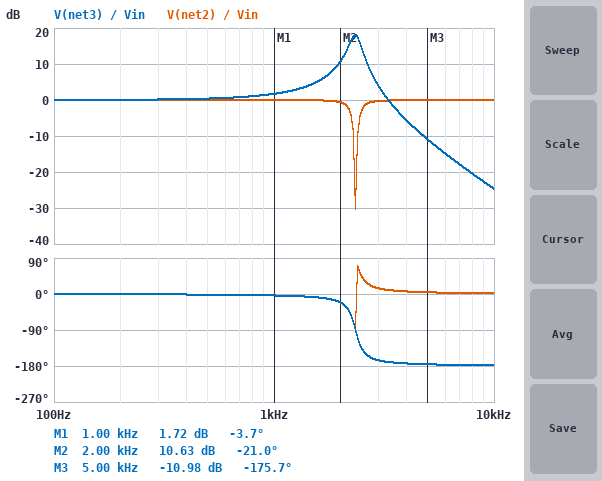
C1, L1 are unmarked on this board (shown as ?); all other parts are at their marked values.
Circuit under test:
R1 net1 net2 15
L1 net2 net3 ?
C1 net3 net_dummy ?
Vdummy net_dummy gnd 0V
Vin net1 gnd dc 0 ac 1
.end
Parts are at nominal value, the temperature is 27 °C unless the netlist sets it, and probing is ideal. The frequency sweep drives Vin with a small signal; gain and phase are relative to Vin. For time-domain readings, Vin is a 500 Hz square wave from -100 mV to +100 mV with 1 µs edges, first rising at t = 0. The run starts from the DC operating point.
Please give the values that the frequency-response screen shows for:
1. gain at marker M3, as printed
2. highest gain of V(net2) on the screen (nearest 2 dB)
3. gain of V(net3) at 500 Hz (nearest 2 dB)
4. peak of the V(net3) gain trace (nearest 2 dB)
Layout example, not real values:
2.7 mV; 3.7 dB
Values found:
-10.98 dB; 0 dB; 0 dB; 18 dB
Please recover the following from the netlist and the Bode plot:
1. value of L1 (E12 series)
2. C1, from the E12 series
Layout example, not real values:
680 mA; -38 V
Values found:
8.2 mH; 560 nF
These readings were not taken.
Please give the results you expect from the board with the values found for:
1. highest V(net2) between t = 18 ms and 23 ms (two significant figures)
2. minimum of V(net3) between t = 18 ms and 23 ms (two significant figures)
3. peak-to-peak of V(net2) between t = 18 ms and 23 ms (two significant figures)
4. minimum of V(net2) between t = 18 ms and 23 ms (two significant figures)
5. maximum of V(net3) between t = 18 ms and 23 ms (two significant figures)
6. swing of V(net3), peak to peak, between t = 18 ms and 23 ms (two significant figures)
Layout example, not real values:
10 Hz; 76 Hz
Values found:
120 mV; -290 mV; 240 mV; -120 mV; 290 mV; 580 mV
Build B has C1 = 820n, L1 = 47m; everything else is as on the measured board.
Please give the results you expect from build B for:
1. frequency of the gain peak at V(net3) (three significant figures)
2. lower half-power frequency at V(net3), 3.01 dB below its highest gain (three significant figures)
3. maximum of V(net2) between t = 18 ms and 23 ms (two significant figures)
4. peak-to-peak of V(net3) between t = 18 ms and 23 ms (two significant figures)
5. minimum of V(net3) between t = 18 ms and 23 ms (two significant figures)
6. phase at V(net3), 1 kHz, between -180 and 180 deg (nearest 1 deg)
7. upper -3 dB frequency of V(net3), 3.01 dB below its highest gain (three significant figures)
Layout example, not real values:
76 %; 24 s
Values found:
810 Hz; 784 Hz; 110 mV; 440 mV; -220 mV; -172 deg; 835 Hz
